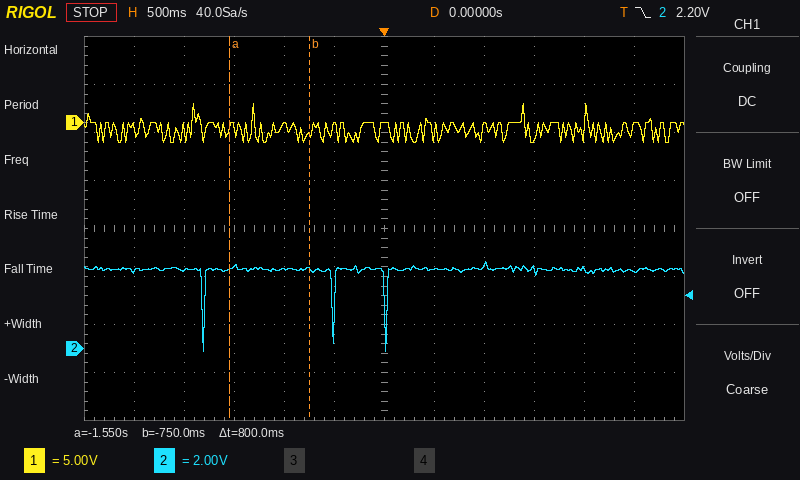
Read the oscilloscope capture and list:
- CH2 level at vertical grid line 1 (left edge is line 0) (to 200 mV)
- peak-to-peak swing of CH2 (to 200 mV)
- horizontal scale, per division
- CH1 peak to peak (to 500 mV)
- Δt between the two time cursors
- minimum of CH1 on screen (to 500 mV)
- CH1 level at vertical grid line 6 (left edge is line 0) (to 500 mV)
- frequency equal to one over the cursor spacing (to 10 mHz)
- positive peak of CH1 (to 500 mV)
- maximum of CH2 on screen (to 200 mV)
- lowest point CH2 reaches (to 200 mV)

3.2 V
3.8 V
500 ms
4.0 V
800 ms
-2.0 V
0.0 V
1.25 Hz
2.0 V
3.6 V
-200 mV
